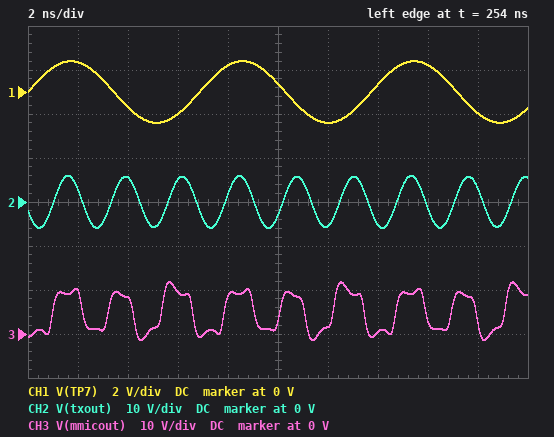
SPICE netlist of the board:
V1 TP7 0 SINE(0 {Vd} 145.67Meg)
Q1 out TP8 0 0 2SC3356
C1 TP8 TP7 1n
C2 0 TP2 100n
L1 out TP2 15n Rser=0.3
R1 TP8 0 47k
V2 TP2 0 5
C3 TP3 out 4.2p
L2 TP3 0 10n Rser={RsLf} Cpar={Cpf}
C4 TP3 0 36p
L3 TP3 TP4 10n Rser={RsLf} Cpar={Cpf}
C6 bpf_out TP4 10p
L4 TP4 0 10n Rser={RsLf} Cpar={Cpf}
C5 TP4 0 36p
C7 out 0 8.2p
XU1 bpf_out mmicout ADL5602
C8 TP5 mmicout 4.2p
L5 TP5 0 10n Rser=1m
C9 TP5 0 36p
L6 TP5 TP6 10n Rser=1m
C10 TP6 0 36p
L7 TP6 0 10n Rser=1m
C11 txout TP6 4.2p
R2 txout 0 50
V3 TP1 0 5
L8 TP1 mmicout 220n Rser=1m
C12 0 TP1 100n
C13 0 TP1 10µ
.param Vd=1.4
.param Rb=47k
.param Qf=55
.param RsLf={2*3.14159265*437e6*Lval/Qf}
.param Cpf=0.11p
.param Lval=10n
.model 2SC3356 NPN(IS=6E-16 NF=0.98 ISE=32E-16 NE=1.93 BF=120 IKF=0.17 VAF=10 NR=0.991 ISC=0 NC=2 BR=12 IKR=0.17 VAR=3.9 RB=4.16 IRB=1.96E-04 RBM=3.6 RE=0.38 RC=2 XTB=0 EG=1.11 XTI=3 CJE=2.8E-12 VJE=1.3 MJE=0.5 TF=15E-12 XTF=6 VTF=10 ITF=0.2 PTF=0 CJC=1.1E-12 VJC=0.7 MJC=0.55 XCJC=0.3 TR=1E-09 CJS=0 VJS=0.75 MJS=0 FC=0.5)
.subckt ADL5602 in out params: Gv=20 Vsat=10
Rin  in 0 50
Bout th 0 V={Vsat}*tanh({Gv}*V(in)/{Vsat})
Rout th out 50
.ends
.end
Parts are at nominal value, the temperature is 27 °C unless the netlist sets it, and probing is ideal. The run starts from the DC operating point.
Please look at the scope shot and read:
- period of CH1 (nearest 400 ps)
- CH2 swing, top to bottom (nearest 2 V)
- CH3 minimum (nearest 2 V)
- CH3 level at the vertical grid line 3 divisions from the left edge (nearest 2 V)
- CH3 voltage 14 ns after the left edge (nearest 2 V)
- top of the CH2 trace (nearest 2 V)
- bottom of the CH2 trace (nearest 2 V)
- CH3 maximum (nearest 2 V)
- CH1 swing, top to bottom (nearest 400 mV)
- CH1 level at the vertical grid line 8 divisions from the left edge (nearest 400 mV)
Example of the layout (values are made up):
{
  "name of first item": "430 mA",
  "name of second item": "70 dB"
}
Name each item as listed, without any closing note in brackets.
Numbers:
{
  "period of CH1": "6.8 ns",
  "CH2 swing, top to bottom": "12 V",
  "CH3 minimum": "-2 V",
  "CH3 level at the vertical grid line 3 divisions from the left edge": "10 V",
  "CH3 voltage 14 ns after the left edge": "0 V",
  "top of the CH2 trace": "6 V",
  "bottom of the CH2 trace": "-6 V",
  "CH3 maximum": "12 V",
  "CH1 swing, top to bottom": "2.8 V",
  "CH1 level at the vertical grid line 8 divisions from the left edge": "1.2 V"
}
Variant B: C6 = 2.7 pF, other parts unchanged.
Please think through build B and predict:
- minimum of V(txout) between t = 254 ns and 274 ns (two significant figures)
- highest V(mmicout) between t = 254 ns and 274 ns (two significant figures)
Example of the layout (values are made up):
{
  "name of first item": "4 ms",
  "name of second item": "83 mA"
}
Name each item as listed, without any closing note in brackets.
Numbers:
{
  "minimum of V(txout) between t = 254 ns and 274 ns": "-5.6 V",
  "highest V(mmicout) between t = 254 ns and 274 ns": "11 V"
}
